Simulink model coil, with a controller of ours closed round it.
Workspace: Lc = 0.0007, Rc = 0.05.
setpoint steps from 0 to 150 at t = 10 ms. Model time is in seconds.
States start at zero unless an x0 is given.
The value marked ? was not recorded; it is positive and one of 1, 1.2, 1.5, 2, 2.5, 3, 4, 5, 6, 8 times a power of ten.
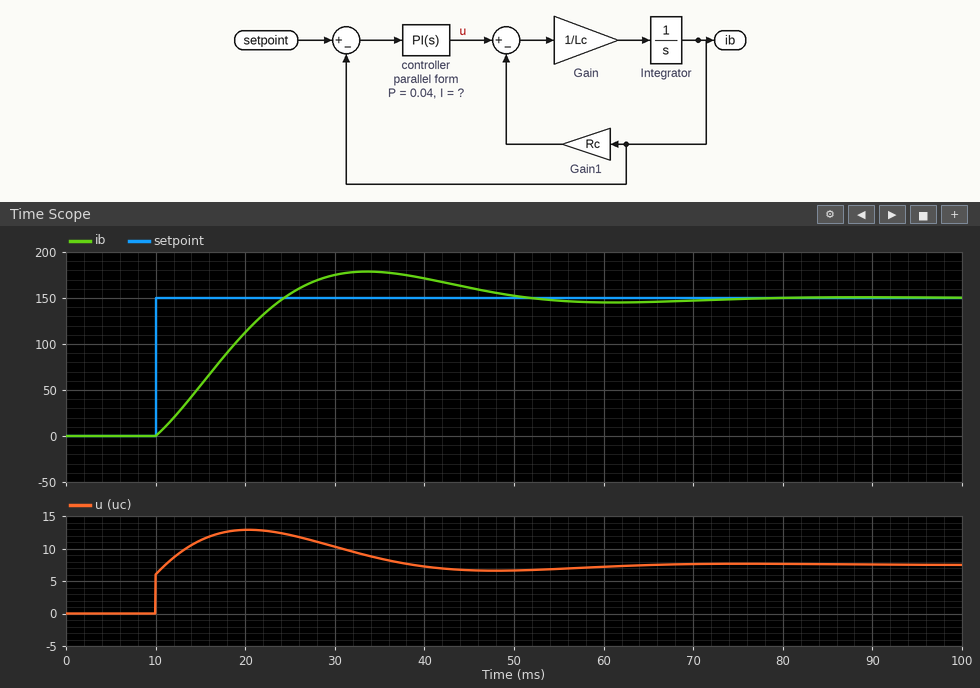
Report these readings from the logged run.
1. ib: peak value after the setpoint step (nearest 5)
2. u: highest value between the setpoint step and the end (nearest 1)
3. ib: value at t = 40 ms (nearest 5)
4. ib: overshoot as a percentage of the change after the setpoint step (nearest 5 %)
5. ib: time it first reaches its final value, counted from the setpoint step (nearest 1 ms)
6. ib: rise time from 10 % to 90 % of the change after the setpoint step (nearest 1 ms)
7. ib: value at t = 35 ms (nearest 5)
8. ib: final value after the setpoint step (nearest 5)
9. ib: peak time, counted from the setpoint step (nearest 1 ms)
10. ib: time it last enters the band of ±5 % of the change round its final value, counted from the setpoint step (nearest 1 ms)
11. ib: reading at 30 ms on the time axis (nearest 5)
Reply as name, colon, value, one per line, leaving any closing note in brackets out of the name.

ib: peak value after the setpoint step: 180
u: highest value between the setpoint step and the end: 13
ib: value at t = 40 ms: 170
ib: overshoot as a percentage of the change after the setpoint step: 20 %
ib: time it first reaches its final value, counted from the setpoint step: 14 ms
ib: rise time from 10 % to 90 % of the change after the setpoint step: 11 ms
ib: value at t = 35 ms: 180
ib: final value after the setpoint step: 150
ib: peak time, counted from the setpoint step: 24 ms
ib: time it last enters the band of ±5 % of the change round its final value, counted from the setpoint step: 37 ms
ib: reading at 30 ms on the time axis: 175
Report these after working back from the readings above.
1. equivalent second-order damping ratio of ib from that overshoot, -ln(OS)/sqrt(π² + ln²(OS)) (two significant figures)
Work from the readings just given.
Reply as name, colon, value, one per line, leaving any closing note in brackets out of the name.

equivalent second-order damping ratio of ib from that overshoot, -ln(OS)/sqrt(π² + ln²(OS)): 0.46
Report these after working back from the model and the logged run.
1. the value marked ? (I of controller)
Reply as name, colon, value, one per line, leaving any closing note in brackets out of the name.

the value marked ?: 12
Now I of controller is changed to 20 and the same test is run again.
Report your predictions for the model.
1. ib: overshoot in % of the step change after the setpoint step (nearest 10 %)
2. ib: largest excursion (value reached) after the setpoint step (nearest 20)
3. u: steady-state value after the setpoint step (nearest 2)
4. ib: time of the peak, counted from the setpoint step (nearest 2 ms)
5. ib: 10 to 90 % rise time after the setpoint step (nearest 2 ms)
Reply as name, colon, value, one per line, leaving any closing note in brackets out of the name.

ib: overshoot in % of the step change after the setpoint step: 30 %
ib: largest excursion (value reached) after the setpoint step: 200
u: steady-state value after the setpoint step: 8
ib: time of the peak, counted from the setpoint step: 18 ms
ib: 10 to 90 % rise time after the setpoint step: 8 ms
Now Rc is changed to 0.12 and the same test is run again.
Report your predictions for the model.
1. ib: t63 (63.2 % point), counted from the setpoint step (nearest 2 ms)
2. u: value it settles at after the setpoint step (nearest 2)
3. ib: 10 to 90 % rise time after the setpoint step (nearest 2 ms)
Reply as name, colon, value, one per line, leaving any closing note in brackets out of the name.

ib: t63 (63.2 % point), counted from the setpoint step: 12 ms
u: value it settles at after the setpoint step: 18
ib: 10 to 90 % rise time after the setpoint step: 20 ms
